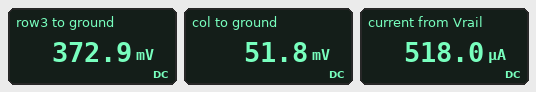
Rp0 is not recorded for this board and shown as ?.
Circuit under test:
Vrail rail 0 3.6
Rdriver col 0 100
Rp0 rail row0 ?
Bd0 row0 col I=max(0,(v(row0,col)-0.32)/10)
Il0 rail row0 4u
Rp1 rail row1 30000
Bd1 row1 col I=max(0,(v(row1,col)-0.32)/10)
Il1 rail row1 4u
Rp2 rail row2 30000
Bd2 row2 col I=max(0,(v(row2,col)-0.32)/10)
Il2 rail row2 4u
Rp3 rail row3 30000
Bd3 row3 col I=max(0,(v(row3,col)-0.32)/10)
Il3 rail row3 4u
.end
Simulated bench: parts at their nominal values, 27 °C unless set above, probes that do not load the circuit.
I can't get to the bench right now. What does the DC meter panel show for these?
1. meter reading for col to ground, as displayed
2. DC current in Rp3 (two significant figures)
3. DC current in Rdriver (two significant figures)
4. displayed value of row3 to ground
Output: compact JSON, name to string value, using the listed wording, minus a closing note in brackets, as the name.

{"meter reading for col to ground, as displayed": "51.8 mV", "DC current in Rp3": "110 µA", "DC current in Rdriver": "520 µA", "displayed value of row3 to ground": "372.9 mV"}
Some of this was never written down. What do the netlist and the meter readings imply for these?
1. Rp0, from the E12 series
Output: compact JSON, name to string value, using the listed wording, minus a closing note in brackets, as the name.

{"Rp0, from the E12 series": "18 kΩ"}
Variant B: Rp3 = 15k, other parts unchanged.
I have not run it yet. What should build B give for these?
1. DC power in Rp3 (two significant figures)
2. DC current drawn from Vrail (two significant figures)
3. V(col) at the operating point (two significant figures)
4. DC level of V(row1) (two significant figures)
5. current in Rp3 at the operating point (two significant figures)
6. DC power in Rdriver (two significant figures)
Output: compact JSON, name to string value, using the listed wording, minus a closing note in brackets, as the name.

{"DC power in Rp3": "690 µW", "DC current drawn from Vrail": "620 µA", "V(col) at the operating point": "62 mV", "DC level of V(row1)": "380 mV", "current in Rp3 at the operating point": "210 µA", "DC power in Rdriver": "39 µW"}
